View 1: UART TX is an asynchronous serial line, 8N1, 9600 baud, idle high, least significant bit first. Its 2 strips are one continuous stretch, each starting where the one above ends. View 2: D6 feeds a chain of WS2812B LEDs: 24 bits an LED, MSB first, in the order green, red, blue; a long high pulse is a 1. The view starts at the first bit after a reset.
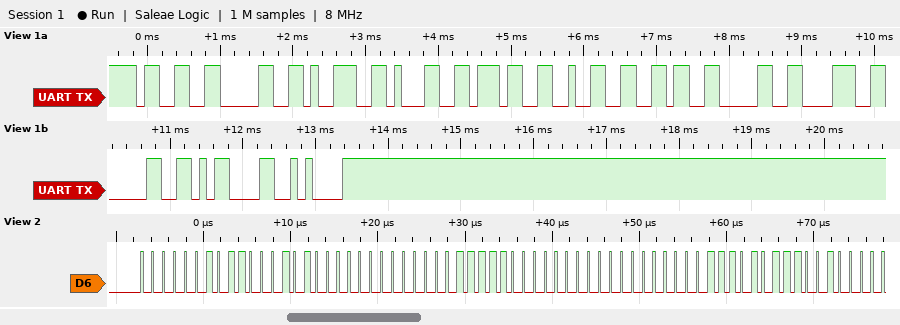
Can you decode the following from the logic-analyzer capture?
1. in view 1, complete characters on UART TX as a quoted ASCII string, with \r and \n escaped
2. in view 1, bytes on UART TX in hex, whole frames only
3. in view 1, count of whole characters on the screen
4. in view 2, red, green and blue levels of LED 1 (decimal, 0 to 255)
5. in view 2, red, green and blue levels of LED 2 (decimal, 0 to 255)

"3091726080\r\n"
33 30 39 31 37 32 36 30 38 30 0D 0A
12
197, 2, 0
192, 7, 0
